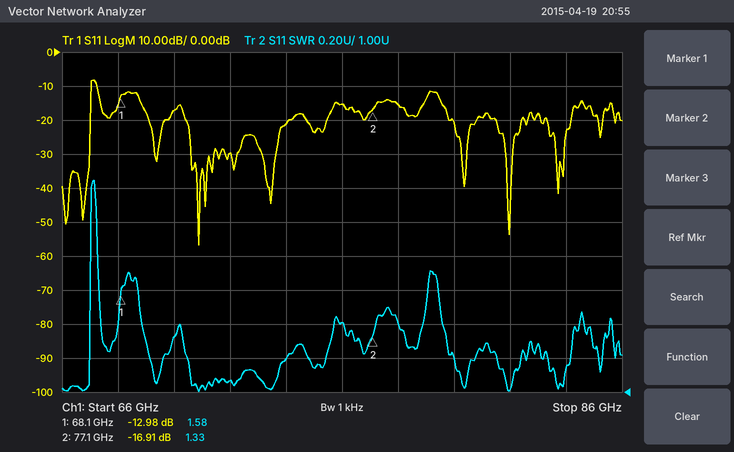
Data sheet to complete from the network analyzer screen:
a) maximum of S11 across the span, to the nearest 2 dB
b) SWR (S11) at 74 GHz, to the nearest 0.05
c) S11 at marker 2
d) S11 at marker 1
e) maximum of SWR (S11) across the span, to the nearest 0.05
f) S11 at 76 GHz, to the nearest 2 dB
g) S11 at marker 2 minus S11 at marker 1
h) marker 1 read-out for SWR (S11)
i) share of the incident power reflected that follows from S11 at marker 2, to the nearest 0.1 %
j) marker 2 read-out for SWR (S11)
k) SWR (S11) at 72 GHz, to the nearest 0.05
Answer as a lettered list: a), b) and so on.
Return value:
a) -8 dB
b) 1.20
c) -16.91 dB
d) -12.98 dB
e) 2.25
f) -16 dB
g) -3.93 dB
h) 1.58
i) 2.0 %
j) 1.33
k) 1.05
